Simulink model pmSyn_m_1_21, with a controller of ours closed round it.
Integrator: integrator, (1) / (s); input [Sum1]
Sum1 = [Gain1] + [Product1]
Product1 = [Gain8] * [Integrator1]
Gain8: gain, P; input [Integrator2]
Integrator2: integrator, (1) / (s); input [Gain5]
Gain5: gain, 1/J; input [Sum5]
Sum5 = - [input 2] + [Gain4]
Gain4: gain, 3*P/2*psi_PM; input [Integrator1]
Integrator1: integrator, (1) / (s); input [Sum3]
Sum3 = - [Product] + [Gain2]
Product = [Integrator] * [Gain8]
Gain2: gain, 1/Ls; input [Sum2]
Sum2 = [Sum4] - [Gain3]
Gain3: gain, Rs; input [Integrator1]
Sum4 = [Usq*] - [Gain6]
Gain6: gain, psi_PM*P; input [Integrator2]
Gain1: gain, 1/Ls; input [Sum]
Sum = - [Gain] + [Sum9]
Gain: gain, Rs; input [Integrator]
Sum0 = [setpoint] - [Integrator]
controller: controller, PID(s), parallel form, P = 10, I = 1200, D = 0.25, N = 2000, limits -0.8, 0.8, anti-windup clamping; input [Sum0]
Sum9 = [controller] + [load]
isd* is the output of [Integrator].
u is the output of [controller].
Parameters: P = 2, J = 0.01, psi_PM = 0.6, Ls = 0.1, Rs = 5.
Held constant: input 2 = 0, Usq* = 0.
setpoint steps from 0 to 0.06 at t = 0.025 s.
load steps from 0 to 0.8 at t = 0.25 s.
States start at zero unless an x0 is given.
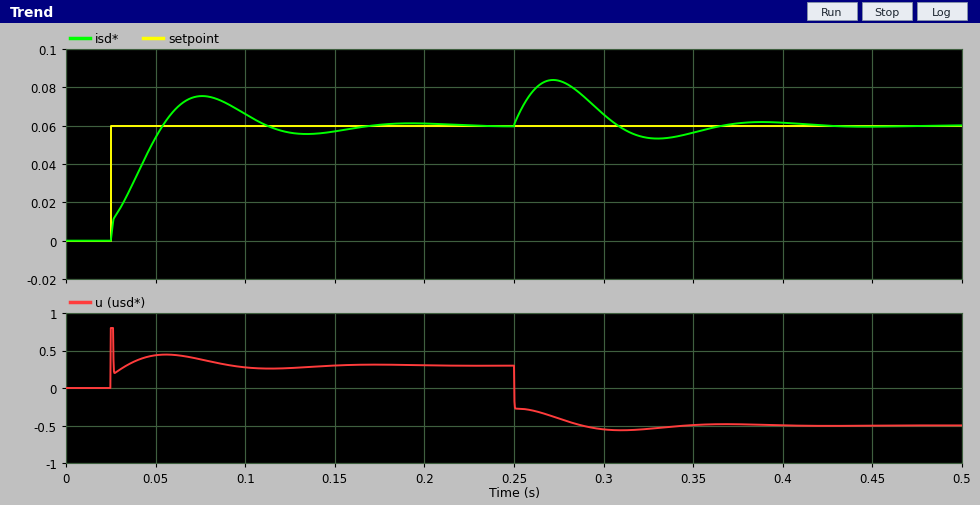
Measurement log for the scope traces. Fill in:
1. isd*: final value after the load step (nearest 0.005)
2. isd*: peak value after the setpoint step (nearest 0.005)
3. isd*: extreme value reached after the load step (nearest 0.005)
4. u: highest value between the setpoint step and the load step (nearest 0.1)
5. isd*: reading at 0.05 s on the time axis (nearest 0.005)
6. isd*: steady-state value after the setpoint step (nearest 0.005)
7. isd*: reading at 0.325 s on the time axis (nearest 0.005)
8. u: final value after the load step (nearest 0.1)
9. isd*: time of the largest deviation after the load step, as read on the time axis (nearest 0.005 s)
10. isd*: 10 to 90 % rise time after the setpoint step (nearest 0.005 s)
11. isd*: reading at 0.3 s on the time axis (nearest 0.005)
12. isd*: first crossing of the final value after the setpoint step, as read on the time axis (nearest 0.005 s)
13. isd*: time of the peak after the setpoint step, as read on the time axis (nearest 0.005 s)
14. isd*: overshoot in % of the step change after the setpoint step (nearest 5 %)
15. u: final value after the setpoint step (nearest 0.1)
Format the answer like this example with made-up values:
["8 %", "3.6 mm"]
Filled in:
["0.060", "0.075", "0.085", "0.8", "0.055", "0.060", "0.055", "-0.5", "0.270 s", "0.025 s", "0.065", "0.055 s", "0.075 s", "25 %", "0.3"]
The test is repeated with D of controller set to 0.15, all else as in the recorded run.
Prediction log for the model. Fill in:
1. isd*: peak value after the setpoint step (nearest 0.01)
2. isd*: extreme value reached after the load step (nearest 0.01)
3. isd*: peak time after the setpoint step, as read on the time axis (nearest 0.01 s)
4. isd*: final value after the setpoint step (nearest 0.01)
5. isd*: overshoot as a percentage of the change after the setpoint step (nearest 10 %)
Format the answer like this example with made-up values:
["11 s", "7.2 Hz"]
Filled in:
["0.07", "0.09", "0.07 s", "0.06", "20 %"]
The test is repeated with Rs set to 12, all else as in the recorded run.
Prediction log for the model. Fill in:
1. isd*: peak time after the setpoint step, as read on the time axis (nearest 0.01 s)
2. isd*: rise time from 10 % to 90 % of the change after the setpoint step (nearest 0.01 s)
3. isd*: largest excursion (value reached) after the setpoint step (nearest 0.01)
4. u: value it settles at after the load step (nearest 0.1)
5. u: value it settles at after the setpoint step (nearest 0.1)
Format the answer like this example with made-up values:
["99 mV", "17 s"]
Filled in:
["0.09 s", "0.03 s", "0.07", "-0.1", "0.7"]
